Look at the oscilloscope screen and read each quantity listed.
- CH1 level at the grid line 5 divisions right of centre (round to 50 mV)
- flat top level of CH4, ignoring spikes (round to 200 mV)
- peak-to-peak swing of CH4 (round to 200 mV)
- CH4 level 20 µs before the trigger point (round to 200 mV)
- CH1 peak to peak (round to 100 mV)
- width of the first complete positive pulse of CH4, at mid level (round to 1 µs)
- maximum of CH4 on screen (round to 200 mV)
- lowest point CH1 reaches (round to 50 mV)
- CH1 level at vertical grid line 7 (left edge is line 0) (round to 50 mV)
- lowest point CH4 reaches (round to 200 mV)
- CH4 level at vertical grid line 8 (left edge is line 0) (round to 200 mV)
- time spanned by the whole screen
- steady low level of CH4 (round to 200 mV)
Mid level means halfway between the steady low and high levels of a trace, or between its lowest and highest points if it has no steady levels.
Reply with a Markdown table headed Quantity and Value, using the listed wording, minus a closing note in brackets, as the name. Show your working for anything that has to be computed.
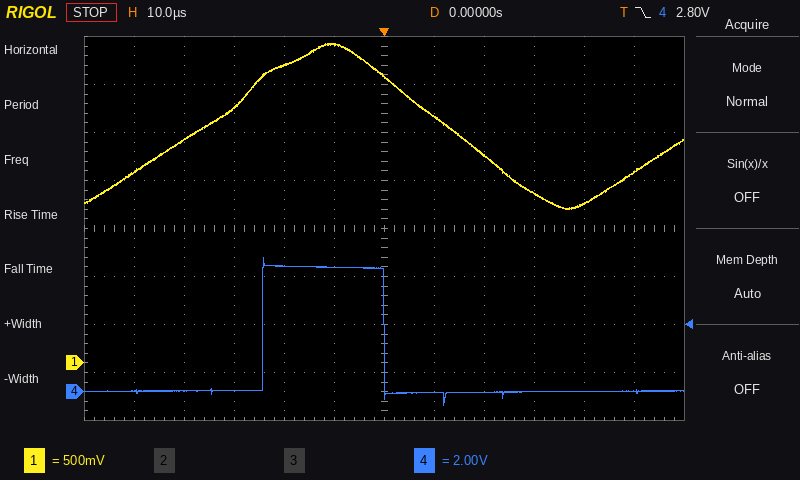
| Quantity | Value |
|---|---|
| CH1 level at the grid line 5 divisions right of centre | 2.00 V |
| flat top level of CH4, ignoring spikes | 5.2 V |
| peak-to-peak swing of CH4 | 5.6 V − (-600 mV) = 6.2 V |
| CH4 level 20 µs before the trigger point | 5.2 V |
| CH1 peak to peak | 1.70 V |
| width of the first complete positive pulse of CH4, at mid level | 24 µs |
| maximum of CH4 on screen | 5.6 V |
| lowest point CH1 reaches | 1.60 V |
| CH1 level at vertical grid line 7 (left edge is line 0) | 2.55 V |
| lowest point CH4 reaches | -600 mV |
| CH4 level at vertical grid line 8 (left edge is line 0) | 0.0 V |
| time spanned by the whole screen | 120 µs |
| steady low level of CH4 | 0.0 V |
